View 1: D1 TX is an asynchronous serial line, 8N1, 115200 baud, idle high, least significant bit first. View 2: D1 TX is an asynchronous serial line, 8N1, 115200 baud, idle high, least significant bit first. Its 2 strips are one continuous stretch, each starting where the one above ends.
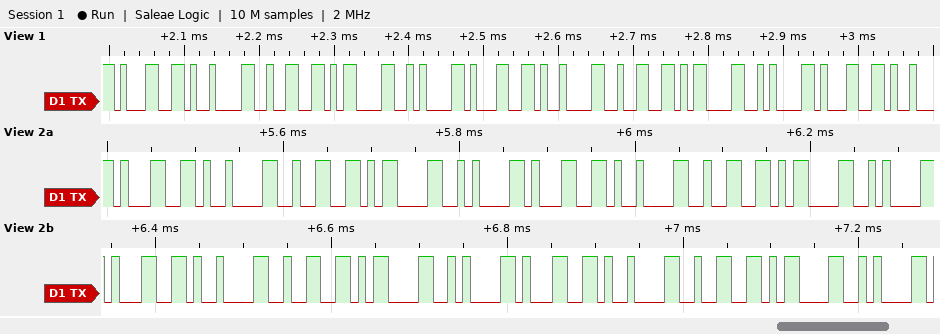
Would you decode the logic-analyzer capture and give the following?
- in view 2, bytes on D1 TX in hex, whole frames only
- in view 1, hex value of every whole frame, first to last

31 09 32 0D 0A 31 09 32 0D 0A 31 09 32 0D 0A 31 09 32 0D 0A
31 09 32 0D 0A 31 09 32 0D 0A 31
